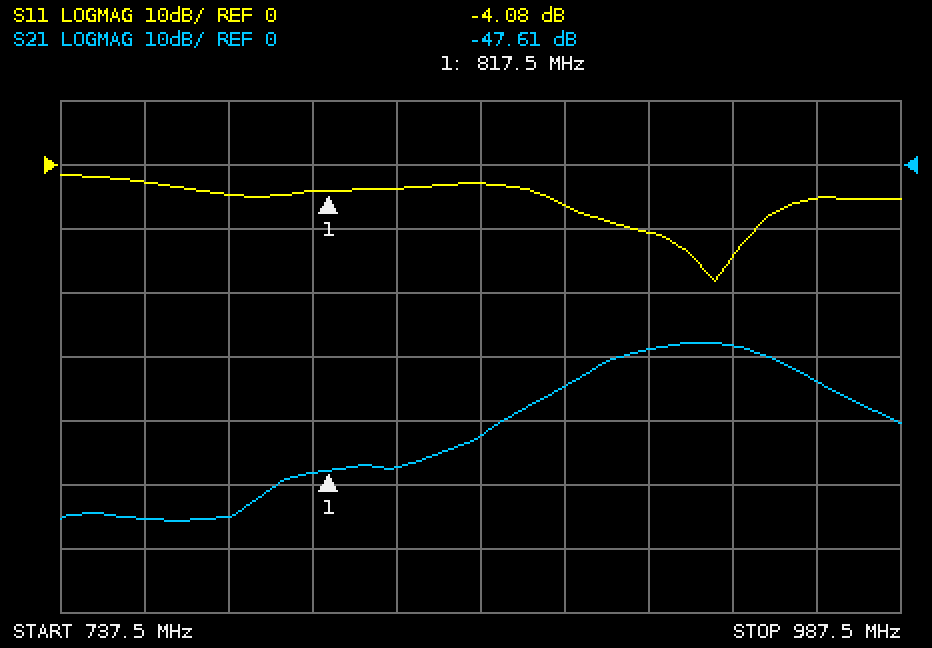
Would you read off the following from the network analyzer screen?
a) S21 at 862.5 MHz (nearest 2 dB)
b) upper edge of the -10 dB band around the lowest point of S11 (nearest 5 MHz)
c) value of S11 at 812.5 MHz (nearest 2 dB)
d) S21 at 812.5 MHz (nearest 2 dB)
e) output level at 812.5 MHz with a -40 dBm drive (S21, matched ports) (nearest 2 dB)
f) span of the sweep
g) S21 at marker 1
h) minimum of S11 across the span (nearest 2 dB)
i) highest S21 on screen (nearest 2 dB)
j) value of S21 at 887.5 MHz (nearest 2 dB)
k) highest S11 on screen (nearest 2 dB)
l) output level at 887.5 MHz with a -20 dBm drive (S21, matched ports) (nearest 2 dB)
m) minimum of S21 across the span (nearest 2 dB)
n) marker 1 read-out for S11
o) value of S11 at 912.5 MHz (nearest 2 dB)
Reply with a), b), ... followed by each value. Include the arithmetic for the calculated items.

a) -42 dB
b) 945 MHz
c) -4 dB
d) -48 dB
e) -40 dBm + (-48 dB) = -88 dBm
f) 250 MHz
g) -47.61 dB
h) -18 dB
i) -28 dB
j) -34 dB
k) -2 dB
l) -20 dBm + (-34 dB) = -54 dBm
m) -56 dB
n) -4.08 dB
o) -10 dB
